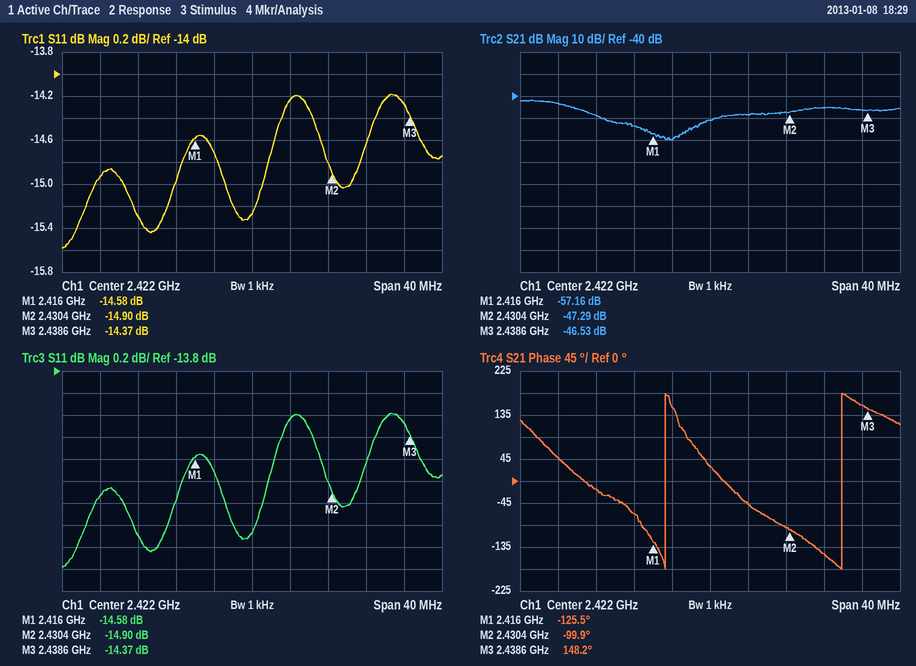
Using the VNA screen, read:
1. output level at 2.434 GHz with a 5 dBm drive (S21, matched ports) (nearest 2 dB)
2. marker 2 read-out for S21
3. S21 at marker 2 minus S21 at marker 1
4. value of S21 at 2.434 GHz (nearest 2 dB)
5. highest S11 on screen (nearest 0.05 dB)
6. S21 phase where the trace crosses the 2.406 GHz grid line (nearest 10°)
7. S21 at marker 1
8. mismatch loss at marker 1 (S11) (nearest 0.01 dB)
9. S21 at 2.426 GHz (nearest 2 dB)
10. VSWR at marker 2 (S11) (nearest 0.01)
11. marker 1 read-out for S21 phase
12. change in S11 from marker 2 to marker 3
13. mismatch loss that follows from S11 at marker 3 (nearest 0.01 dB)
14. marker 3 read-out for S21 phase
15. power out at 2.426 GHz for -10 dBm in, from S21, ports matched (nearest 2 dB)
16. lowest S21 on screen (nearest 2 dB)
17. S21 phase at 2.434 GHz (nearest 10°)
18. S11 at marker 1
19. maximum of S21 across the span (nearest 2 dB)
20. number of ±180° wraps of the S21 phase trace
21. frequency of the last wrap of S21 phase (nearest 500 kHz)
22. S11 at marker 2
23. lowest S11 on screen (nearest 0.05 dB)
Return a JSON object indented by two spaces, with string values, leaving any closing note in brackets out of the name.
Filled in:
{
  "output level at 2.434 GHz with a 5 dBm drive (S21, matched ports)": "-40 dBm",
  "marker 2 read-out for S21": "-47.29 dB",
  "S21 at marker 2 minus S21 at marker 1": "9.87 dB",
  "value of S21 at 2.434 GHz": "-46 dB",
  "highest S11 on screen": "-14.20 dB",
  "S21 phase where the trace crosses the 2.406 GHz grid line": "50°",
  "S21 at marker 1": "-57.16 dB",
  "mismatch loss at marker 1 (S11)": "0.15 dB",
  "S21 at 2.426 GHz": "-48 dB",
  "VSWR at marker 2 (S11)": "1.44",
  "marker 1 read-out for S21 phase": "-125.5°",
  "change in S11 from marker 2 to marker 3": "0.53 dB",
  "mismatch loss that follows from S11 at marker 3": "0.16 dB",
  "marker 3 read-out for S21 phase": "148.2°",
  "power out at 2.426 GHz for -10 dBm in, from S21, ports matched": "-58 dBm",
  "lowest S21 on screen": "-60 dB",
  "S21 phase at 2.434 GHz": "-150°",
  "S11 at marker 1": "-14.58 dB",
  "maximum of S21 across the span": "-42 dB",
  "number of ±180° wraps of the S21 phase trace": "2",
  "frequency of the last wrap of S21 phase": "2.4360 GHz",
  "S11 at marker 2": "-14.90 dB",
  "lowest S11 on screen": "-15.60 dB"
}
